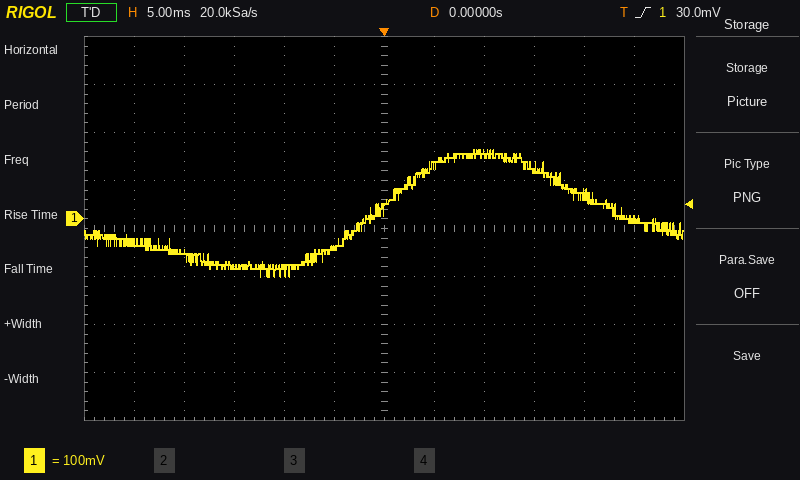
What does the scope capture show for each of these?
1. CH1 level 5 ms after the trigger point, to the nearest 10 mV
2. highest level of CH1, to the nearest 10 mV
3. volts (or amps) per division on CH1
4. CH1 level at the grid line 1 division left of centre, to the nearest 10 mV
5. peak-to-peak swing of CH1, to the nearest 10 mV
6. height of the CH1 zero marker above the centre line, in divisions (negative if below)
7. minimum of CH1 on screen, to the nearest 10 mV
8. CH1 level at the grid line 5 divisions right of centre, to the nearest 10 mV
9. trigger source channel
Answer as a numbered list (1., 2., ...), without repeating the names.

1. 110 mV
2. 140 mV
3. 100 mV
4. -60 mV
5. 260 mV
6. +0.2 div
7. -120 mV
8. 0 mV
9. CH1
